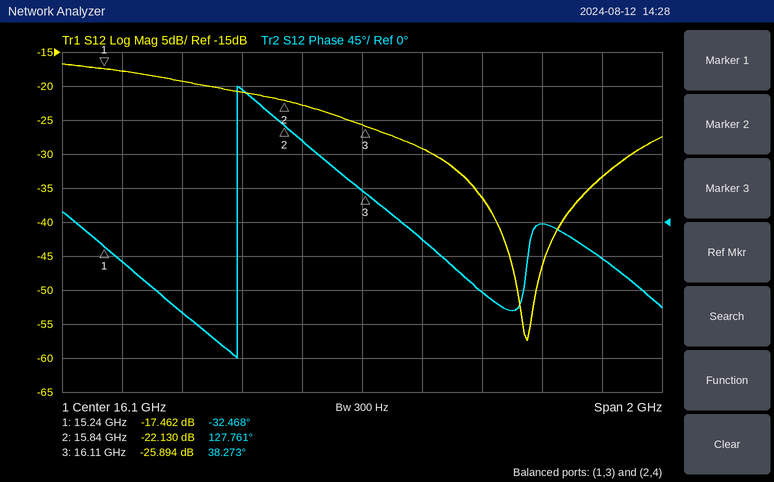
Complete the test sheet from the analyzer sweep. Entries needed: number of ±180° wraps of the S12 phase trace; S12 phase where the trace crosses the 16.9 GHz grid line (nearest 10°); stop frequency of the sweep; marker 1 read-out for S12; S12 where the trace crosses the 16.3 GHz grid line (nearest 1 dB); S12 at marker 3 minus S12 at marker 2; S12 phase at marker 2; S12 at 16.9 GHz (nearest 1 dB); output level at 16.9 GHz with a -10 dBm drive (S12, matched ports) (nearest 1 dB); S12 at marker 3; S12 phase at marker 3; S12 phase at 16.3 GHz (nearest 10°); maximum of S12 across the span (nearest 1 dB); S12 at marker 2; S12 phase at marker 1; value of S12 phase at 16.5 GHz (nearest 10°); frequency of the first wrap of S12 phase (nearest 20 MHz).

1
-50°
17.1 GHz
-17.462 dB
-29 dB
-3.764 dB
127.761°
-33 dB
-43 dBm
-25.894 dB
38.273°
-20°
-17 dB
-22.130 dB
-32.468°
-90°
15.68 GHz
